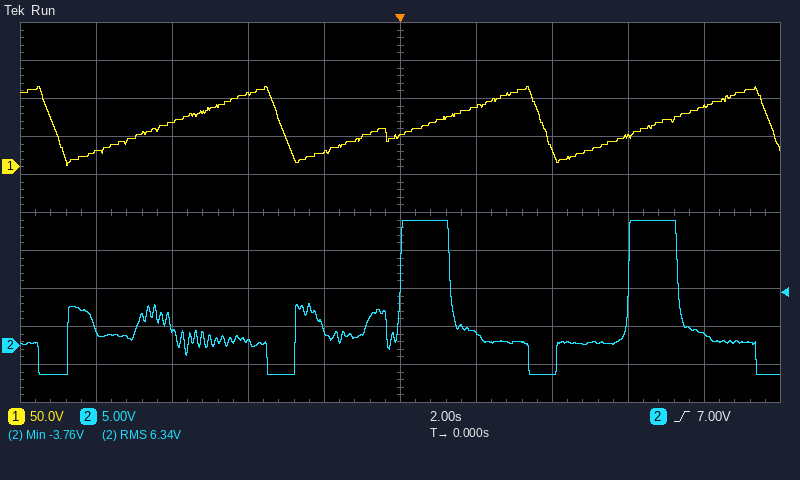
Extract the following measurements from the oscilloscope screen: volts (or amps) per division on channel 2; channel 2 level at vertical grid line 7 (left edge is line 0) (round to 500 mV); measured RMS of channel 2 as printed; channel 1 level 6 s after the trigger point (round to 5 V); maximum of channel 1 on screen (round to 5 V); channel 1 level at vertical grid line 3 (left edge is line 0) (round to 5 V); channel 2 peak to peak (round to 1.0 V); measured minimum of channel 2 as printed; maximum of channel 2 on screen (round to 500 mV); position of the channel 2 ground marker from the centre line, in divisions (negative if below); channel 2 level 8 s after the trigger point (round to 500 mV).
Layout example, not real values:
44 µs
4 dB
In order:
5 V
-3.5 V
6.34 V
40 V
105 V
95 V
20.0 V
-3.76 V
16.5 V
-3.5 div
1.5 V
